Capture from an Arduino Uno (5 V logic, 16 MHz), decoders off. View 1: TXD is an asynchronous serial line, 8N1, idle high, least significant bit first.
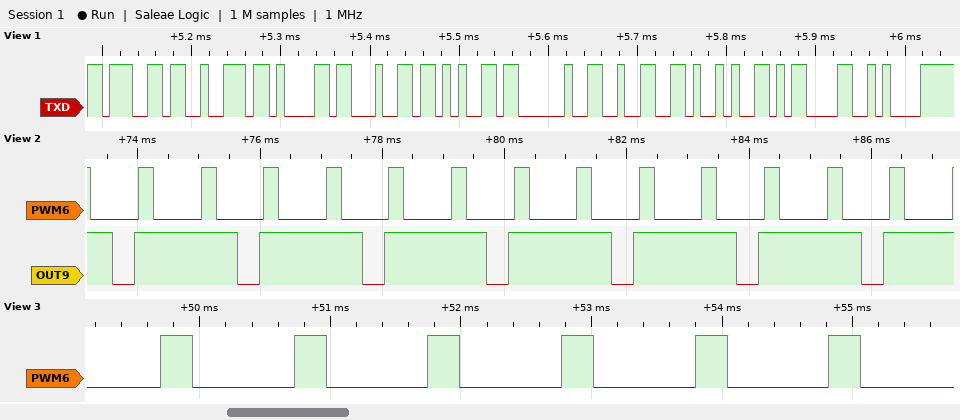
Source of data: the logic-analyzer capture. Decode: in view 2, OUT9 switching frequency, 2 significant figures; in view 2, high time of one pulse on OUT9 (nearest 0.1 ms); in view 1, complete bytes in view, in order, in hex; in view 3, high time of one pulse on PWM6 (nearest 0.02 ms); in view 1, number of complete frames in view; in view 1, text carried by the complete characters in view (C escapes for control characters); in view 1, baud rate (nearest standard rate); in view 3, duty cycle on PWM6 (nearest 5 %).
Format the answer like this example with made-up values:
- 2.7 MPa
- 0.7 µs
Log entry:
- 490 Hz
- 1.7 ms
- 67 72 61 64 65 20 32 29 0D 0A
- 0.24 ms
- 10
- "grade 2)\r\n"
- 115200 baud
- 25 %
